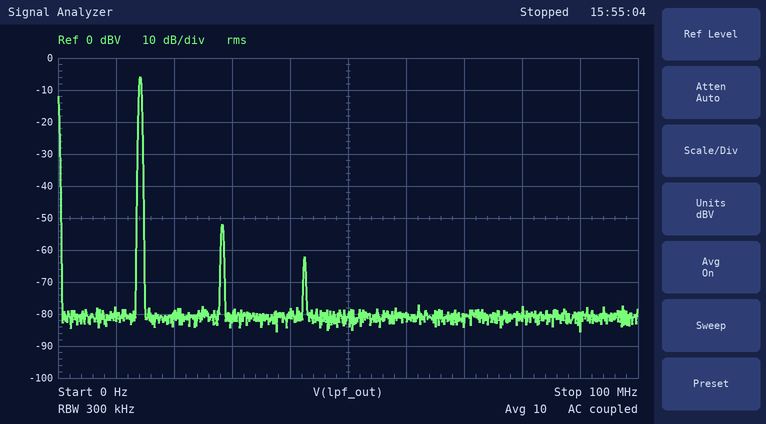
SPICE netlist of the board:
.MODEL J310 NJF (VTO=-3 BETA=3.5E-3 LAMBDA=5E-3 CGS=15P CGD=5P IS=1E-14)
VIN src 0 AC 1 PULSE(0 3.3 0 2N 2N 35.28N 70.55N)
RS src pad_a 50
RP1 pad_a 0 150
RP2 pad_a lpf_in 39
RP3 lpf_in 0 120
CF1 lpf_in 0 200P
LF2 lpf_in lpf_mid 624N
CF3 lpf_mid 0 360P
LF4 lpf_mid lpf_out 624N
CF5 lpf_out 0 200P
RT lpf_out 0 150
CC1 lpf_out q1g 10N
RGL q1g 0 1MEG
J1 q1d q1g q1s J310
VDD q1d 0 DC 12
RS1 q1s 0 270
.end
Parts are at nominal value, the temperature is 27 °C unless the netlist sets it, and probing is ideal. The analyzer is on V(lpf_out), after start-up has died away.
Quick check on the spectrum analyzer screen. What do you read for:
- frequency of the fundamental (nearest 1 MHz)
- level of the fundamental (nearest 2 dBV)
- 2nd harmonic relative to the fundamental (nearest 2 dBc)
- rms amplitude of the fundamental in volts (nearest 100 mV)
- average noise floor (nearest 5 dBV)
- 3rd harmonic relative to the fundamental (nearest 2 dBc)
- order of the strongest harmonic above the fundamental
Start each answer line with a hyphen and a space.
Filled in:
- 14 MHz
- -6 dBV
- -46 dBc
- 500 mV
- -80 dBV
- -56 dBc
- 2
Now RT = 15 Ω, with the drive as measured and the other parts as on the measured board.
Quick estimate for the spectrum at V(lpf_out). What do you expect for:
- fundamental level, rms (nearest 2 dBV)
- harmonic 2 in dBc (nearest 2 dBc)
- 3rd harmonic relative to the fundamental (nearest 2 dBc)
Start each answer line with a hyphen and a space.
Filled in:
- -16 dBV
- -44 dBc
- -50 dBc
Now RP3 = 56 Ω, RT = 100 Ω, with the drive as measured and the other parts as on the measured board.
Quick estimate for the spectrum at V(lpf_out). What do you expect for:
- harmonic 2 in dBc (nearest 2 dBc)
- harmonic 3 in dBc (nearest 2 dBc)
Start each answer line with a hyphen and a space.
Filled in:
- -44 dBc
- -54 dBc
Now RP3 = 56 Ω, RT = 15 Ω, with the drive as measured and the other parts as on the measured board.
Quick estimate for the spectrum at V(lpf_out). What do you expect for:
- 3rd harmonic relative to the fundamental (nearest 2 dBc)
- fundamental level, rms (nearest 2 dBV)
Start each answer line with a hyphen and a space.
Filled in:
- -50 dBc
- -16 dBV
